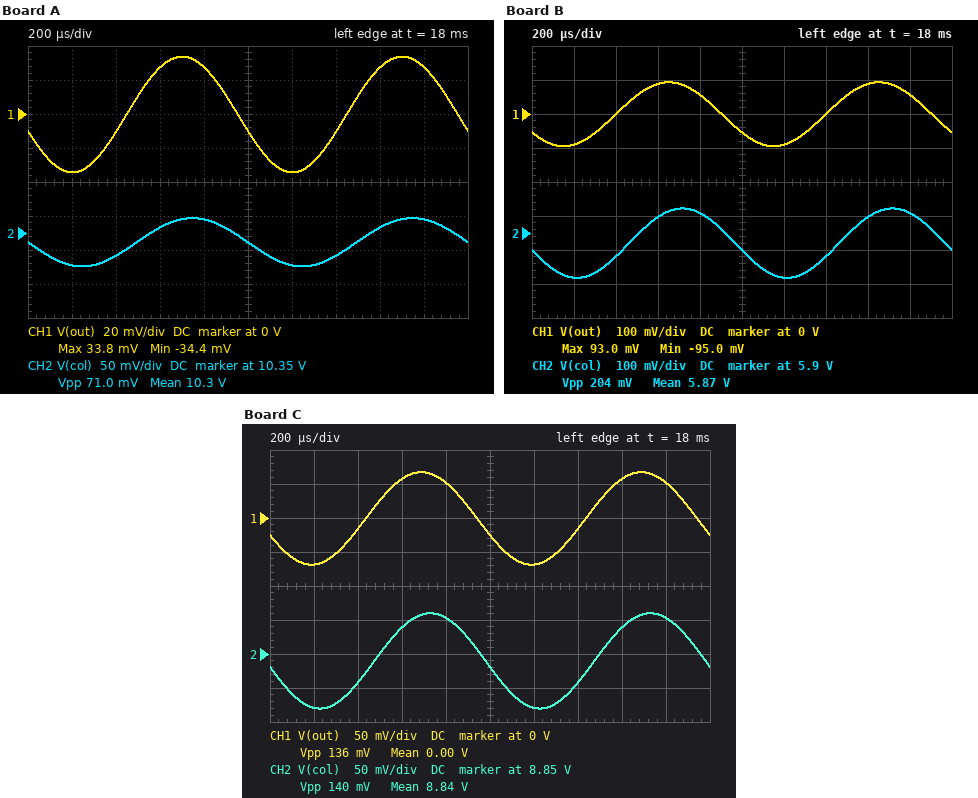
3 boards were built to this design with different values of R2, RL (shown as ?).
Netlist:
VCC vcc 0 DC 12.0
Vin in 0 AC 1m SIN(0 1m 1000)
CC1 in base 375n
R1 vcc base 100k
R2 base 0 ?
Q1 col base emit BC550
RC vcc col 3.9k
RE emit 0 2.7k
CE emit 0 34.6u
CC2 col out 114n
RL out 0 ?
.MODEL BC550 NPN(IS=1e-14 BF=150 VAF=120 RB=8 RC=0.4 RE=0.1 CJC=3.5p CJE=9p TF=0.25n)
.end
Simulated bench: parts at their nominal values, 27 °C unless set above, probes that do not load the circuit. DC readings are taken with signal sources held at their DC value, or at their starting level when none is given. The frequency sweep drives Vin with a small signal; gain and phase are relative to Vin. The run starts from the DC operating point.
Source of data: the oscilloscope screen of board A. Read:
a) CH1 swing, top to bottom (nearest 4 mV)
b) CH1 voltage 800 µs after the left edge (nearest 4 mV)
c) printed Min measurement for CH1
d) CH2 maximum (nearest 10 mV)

68 mV
28 mV
-34.4 mV
10.37 V
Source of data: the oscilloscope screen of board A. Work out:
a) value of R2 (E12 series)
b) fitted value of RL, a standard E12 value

18 kΩ
4.7 kΩ
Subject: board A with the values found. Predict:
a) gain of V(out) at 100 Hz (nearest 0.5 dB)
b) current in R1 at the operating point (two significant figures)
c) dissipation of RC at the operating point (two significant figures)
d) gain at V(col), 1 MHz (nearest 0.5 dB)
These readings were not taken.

20.5 dB
100 µA
710 µW
31.0 dB
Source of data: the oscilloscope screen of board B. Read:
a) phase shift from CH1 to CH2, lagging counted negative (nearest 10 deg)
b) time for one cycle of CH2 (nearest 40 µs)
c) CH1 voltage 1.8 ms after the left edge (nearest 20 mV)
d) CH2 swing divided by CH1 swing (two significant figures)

-20 deg
1.00 ms
60 mV
1.1
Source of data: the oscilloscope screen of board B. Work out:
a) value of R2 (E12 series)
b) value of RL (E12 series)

82 kΩ
3.3 kΩ
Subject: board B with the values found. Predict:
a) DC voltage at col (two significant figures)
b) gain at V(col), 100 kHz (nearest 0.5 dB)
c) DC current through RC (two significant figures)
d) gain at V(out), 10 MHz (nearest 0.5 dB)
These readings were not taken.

5.9 V
40.5 dB
1.6 mA
39.5 dB
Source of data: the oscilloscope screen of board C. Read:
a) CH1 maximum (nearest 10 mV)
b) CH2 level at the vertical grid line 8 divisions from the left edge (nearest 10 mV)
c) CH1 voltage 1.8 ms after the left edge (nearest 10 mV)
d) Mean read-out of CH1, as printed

70 mV
8.89 V
50 mV
0.00 V
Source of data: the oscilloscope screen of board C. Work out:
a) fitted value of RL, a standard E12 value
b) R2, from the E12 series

5.6 kΩ
33 kΩ
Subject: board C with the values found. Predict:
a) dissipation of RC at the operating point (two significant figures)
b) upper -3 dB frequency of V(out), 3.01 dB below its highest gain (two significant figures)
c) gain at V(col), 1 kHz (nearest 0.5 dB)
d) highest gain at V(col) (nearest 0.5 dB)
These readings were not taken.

2.6 mW
33 MHz
37.0 dB
37.0 dB
